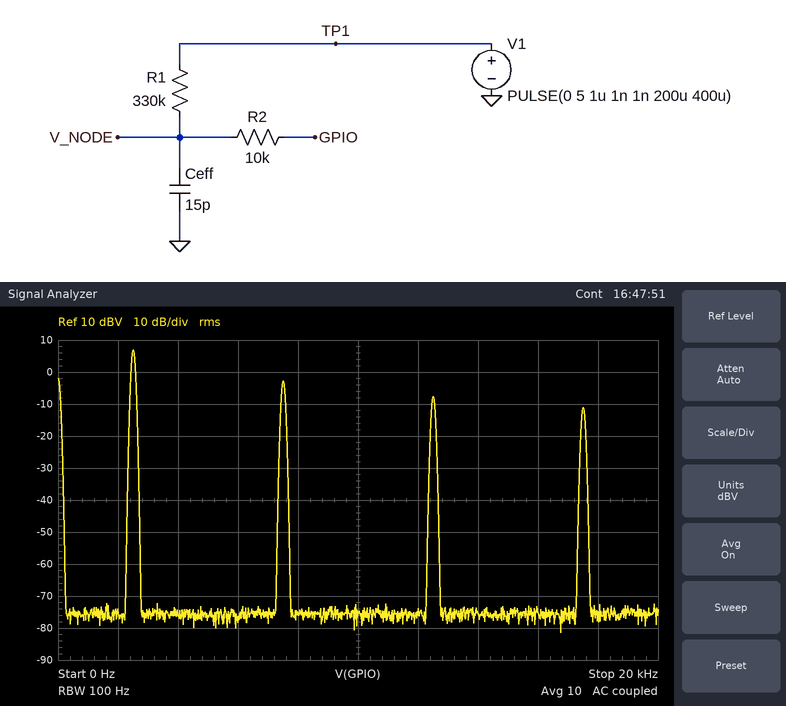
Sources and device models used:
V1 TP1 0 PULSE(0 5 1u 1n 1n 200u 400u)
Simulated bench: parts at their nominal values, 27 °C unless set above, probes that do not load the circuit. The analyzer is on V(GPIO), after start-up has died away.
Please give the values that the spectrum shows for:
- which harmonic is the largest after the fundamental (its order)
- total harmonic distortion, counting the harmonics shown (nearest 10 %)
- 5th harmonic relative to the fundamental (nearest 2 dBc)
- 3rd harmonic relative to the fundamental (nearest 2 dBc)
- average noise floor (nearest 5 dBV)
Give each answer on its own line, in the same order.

3
40 %
-14 dBc
-10 dBc
-75 dBV
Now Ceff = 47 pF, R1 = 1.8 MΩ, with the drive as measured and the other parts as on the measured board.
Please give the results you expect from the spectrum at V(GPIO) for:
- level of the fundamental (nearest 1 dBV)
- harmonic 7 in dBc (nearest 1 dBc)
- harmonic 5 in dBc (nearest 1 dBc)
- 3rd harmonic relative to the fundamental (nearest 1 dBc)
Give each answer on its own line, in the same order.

3 dBV
-32 dBc
-26 dBc
-17 dBc
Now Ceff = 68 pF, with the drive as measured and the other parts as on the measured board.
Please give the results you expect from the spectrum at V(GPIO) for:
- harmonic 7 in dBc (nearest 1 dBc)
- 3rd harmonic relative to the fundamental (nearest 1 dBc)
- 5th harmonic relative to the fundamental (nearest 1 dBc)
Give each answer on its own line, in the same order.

-25 dBc
-12 dBc
-20 dBc
